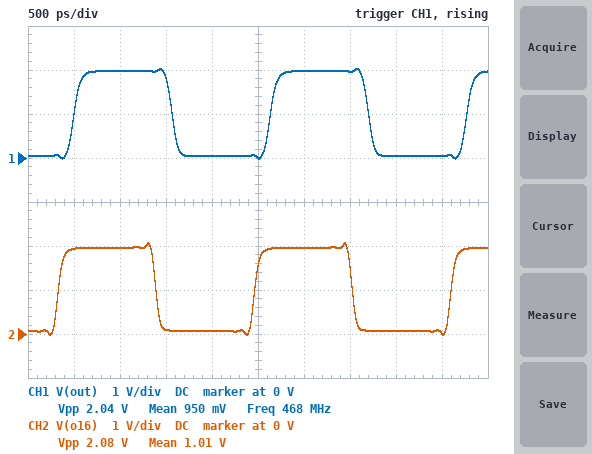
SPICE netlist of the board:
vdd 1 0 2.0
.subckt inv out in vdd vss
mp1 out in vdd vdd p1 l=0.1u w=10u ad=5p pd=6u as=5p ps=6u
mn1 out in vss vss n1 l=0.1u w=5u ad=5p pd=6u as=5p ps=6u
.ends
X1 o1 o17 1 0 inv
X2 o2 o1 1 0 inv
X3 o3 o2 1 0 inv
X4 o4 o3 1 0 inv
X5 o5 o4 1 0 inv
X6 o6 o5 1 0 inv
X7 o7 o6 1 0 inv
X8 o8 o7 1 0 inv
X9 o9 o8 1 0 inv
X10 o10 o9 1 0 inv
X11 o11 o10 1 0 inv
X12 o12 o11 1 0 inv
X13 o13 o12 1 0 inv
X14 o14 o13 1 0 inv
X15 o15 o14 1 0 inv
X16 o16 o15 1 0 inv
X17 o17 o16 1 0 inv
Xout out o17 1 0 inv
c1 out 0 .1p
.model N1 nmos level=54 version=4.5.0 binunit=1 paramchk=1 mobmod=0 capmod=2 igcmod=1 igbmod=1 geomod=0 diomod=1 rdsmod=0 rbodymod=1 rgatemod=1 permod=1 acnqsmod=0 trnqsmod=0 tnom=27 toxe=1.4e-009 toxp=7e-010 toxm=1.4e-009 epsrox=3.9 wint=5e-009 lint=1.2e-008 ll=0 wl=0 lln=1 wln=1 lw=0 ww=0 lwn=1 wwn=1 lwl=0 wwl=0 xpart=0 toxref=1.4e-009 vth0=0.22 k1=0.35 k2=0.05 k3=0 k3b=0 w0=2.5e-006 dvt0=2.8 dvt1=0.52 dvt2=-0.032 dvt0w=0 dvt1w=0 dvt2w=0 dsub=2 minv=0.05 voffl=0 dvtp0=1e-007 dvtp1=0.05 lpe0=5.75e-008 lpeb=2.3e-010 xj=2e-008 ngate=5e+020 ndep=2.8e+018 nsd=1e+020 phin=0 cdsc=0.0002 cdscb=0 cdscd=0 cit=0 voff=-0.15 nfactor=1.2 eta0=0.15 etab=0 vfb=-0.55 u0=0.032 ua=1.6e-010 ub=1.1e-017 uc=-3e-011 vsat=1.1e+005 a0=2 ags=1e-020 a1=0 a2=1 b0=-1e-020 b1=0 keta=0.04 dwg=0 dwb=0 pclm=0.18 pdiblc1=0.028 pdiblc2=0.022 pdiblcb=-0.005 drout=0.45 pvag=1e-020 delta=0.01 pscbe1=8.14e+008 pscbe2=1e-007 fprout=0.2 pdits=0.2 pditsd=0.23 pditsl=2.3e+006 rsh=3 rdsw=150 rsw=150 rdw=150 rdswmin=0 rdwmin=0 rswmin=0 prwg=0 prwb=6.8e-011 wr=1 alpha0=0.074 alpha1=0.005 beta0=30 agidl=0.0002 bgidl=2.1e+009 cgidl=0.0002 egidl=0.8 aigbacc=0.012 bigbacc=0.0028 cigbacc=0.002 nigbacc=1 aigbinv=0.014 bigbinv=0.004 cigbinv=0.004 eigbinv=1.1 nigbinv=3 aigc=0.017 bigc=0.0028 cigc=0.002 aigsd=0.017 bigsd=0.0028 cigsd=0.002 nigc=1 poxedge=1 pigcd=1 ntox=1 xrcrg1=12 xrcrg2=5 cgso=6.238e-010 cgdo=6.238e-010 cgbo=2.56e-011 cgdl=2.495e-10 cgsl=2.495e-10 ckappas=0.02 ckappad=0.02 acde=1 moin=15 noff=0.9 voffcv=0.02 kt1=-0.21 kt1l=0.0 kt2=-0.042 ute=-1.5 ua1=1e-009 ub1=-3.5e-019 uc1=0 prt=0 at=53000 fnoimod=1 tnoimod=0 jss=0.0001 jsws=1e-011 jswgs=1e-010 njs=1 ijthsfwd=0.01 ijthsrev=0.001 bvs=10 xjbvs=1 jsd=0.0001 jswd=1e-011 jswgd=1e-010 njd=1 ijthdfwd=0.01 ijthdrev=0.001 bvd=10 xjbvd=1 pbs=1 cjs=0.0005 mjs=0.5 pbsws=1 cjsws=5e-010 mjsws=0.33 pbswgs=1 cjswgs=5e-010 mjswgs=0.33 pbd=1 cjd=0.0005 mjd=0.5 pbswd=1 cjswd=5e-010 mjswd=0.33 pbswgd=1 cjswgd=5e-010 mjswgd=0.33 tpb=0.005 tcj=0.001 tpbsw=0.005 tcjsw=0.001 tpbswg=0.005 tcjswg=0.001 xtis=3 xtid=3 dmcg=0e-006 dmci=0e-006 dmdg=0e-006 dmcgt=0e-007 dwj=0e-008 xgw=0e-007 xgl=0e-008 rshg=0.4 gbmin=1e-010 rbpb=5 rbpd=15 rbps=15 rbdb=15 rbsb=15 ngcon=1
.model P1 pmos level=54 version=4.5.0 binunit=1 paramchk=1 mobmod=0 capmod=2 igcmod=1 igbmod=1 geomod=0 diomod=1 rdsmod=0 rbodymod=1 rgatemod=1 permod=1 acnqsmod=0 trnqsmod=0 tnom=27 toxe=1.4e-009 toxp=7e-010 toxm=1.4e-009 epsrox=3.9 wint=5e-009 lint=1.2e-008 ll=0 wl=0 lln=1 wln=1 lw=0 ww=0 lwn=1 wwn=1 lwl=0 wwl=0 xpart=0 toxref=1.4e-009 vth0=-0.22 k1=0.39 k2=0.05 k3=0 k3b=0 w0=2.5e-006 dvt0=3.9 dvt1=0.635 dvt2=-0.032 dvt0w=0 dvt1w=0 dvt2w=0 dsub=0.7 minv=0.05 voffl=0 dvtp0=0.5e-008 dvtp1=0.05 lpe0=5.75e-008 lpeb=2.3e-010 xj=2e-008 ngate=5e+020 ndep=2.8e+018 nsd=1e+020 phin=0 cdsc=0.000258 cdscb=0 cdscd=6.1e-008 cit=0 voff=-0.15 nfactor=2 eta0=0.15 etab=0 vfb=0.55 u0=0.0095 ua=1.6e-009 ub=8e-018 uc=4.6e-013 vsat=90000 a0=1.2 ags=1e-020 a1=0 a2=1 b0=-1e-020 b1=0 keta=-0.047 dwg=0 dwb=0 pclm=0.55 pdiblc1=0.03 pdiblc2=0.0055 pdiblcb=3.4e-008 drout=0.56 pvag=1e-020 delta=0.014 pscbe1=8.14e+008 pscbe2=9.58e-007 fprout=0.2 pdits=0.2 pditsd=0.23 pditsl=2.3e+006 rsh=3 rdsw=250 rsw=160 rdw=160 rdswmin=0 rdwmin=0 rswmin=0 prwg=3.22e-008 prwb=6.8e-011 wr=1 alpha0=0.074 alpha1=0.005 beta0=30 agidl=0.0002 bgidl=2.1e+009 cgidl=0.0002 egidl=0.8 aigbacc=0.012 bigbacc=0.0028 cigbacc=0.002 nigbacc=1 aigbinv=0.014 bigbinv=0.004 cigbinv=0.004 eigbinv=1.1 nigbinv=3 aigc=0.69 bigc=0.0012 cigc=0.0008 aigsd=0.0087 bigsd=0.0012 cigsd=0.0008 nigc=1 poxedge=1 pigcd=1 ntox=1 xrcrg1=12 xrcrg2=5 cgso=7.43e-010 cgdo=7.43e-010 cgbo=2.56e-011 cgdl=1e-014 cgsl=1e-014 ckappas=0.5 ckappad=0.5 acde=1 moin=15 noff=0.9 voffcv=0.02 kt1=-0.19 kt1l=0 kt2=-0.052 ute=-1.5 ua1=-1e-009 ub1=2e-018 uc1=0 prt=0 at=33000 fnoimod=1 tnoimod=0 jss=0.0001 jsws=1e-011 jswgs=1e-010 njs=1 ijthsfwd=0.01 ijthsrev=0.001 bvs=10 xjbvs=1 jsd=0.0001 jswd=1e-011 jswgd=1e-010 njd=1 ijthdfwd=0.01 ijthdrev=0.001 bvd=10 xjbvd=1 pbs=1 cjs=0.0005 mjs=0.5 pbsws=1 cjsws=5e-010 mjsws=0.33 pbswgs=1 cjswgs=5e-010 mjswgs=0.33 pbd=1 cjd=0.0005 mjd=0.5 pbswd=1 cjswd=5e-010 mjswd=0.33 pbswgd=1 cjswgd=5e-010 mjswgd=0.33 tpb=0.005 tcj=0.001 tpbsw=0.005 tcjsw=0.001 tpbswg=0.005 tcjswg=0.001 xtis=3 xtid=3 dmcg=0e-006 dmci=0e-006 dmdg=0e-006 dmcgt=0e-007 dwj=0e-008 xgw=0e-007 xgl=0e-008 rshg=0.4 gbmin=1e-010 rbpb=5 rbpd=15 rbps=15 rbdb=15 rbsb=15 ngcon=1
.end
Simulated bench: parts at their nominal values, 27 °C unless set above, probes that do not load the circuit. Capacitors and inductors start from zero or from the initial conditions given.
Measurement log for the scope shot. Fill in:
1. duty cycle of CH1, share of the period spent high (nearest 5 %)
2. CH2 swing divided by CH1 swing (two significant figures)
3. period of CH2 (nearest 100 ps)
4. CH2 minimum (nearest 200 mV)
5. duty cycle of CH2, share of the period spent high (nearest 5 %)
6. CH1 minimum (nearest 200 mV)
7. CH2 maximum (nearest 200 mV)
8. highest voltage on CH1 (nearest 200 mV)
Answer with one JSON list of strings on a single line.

["50 %", "1.0", "2.1 ns", "0 V", "50 %", "0 V", "2.0 V", "2.0 V"]
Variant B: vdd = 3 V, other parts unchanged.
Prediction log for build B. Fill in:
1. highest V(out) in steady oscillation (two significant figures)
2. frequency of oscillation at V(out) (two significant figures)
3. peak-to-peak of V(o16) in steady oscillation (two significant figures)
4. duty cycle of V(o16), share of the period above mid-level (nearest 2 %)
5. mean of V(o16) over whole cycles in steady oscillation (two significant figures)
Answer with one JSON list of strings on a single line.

["2.4 V", "490 MHz", "1.7 V", "50 %", "1.5 V"]
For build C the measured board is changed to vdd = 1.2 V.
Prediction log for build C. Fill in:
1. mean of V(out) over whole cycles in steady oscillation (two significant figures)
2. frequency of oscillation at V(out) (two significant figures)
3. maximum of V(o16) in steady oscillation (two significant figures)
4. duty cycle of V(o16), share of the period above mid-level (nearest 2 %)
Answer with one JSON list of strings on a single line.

["600 mV", "400 MHz", "1.3 V", "50 %"]
